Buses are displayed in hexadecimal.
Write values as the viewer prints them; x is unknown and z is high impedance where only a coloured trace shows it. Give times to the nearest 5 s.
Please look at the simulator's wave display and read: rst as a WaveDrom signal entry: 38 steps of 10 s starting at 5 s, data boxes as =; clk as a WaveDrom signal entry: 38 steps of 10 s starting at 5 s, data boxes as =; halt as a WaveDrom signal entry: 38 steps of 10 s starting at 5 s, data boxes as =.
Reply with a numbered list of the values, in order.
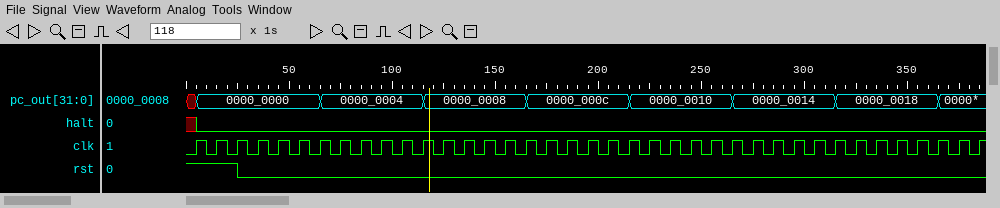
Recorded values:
1. {name: 'rst', wave: '1.0...................................'}
2. {name: 'clk', wave: 'p.....................................'}
3. {name: 'halt', wave: '0.....................................'}
